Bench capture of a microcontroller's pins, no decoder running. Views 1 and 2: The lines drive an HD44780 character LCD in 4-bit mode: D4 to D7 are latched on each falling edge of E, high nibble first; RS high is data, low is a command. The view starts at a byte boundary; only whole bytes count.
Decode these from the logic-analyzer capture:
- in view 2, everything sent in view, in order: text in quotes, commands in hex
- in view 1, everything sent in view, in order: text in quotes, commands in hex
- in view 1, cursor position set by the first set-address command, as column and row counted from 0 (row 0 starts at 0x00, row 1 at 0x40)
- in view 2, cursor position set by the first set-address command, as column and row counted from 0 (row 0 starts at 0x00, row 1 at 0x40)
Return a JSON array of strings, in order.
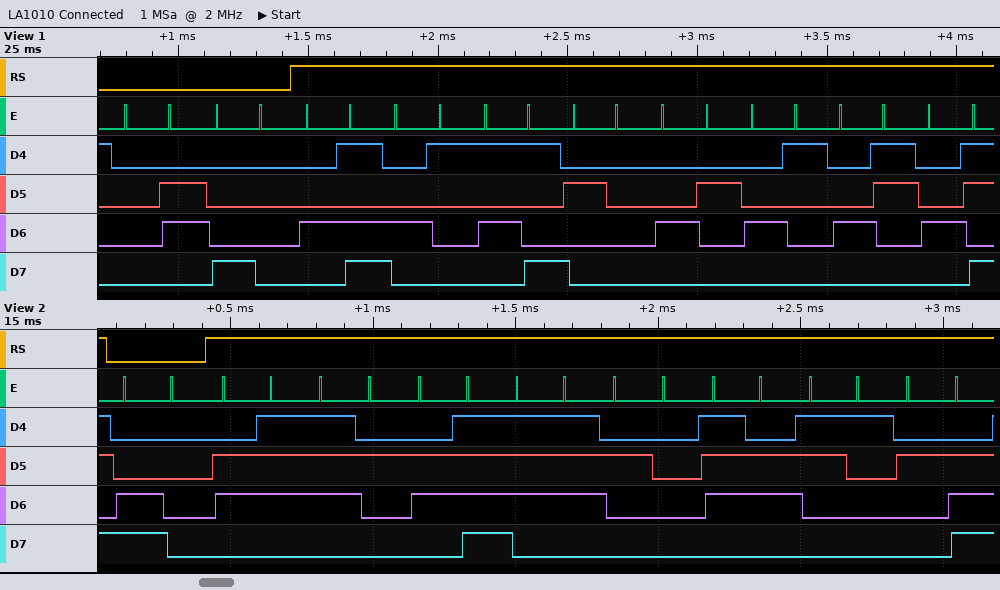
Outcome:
["0xC0 \"grow v1.\"", "0x06 0x80 \"MAY BACK\"", "column 0, row 0", "column 0, row 1"]
